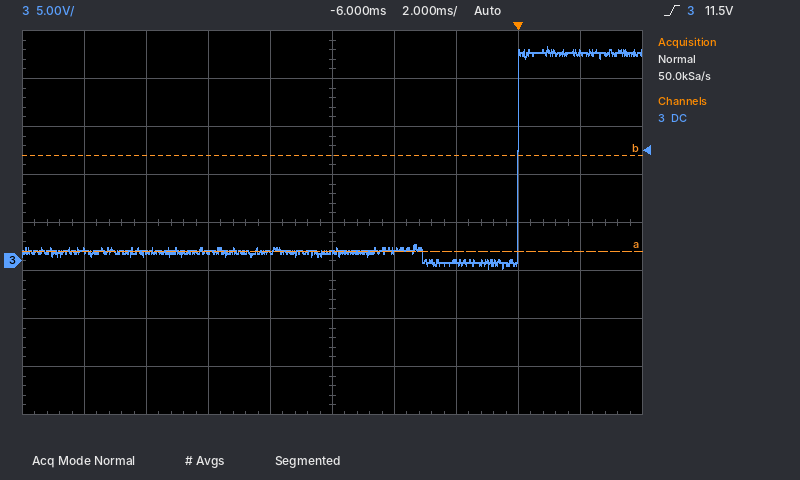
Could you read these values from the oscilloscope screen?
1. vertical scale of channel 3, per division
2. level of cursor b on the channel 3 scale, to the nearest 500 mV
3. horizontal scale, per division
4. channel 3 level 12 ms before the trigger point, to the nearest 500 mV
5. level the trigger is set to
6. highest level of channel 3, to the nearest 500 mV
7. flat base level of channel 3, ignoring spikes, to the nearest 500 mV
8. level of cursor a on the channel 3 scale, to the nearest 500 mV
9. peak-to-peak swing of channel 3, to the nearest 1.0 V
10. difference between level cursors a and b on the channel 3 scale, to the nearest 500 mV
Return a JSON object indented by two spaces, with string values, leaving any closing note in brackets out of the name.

{
  "vertical scale of channel 3, per division": "5 V",
  "level of cursor b on the channel 3 scale, to the nearest 500 mV": "11.0 V",
  "horizontal scale, per division": "2 ms",
  "channel 3 level 12 ms before the trigger point, to the nearest 500 mV": "1.0 V",
  "level the trigger is set to": "11.5 V",
  "highest level of channel 3, to the nearest 500 mV": "22.5 V",
  "flat base level of channel 3, ignoring spikes, to the nearest 500 mV": "1.0 V",
  "level of cursor a on the channel 3 scale, to the nearest 500 mV": "1.0 V",
  "peak-to-peak swing of channel 3, to the nearest 1.0 V": "23.0 V",
  "difference between level cursors a and b on the channel 3 scale, to the nearest 500 mV": "10.0 V"
}
